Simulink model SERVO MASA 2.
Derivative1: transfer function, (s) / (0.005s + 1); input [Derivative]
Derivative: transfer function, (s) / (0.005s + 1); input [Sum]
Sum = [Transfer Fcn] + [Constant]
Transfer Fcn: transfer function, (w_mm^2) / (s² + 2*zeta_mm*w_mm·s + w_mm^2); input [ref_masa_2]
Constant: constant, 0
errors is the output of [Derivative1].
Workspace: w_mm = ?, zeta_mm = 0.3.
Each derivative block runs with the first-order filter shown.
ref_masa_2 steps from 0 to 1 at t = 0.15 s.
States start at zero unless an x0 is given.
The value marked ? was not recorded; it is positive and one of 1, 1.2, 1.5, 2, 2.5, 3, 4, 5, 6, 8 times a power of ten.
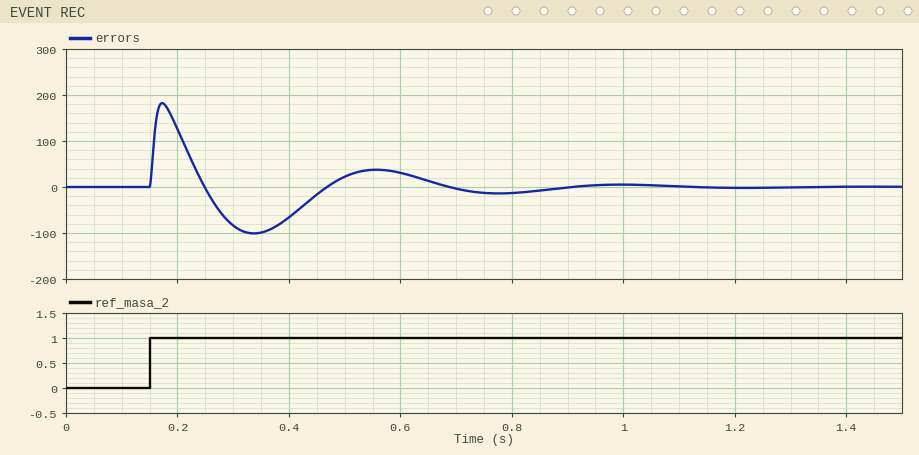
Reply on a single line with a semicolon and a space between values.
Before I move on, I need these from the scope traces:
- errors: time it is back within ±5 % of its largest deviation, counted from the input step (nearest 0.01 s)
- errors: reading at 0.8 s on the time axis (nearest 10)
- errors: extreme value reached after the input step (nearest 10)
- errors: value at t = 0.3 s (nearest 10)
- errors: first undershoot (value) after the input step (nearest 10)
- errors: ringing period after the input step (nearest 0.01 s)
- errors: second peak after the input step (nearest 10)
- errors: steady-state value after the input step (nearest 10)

0.69 s; -10; 180; -80; -100; 0.38 s; 40; 0
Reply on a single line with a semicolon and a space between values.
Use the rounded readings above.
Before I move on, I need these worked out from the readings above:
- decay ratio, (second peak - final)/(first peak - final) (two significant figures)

0.22
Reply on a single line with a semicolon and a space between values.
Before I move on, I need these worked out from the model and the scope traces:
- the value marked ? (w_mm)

15
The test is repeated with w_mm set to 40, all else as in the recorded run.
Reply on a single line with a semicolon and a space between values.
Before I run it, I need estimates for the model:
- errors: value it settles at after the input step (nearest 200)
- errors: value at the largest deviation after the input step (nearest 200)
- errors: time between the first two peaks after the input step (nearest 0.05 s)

0; 1000; 0.15 s
